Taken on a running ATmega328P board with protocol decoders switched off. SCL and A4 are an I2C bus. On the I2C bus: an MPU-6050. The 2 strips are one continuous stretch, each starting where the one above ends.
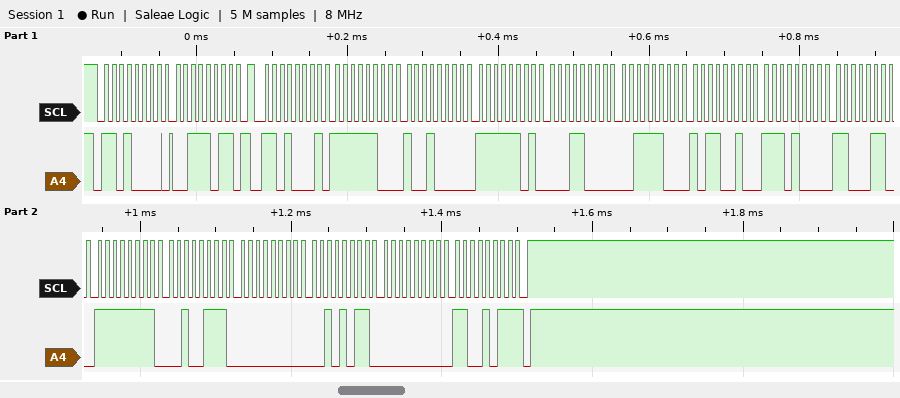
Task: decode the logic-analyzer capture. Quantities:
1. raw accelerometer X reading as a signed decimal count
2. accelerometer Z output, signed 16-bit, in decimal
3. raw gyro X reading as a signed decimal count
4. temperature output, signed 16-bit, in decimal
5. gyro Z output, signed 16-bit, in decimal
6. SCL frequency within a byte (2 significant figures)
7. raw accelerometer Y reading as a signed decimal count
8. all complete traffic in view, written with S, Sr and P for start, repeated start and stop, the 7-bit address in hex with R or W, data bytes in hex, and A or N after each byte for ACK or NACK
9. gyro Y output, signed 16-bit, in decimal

-880
15538
-217
-5946
203
100 kHz
-744
S 68W A 3B A Sr 68R A FC A 90 A FD A 18 A 3C A B2 A E8 A C6 A FF A 27 A 00 A 2B A 00 A CB N P
43
